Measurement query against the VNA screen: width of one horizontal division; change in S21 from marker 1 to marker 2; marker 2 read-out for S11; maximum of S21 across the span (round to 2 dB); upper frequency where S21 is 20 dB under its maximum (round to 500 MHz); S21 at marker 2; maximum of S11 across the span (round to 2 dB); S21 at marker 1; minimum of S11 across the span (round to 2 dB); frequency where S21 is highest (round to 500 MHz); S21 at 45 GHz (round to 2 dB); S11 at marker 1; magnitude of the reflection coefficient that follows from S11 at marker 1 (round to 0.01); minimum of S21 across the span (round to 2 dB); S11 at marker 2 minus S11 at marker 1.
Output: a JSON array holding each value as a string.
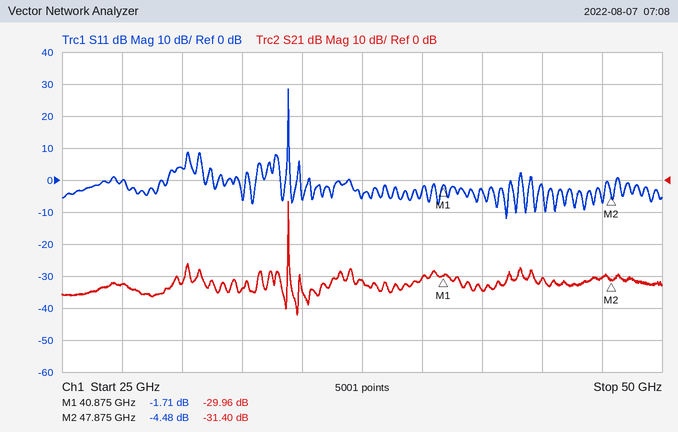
["2.5 GHz", "-1.44 dB", "-4.48 dB", "-6 dB", "34.5 GHz", "-31.40 dB", "28 dB", "-29.96 dB", "-12 dB", "34.5 GHz", "-30 dB", "-1.71 dB", "0.82", "-42 dB", "-2.77 dB"]
